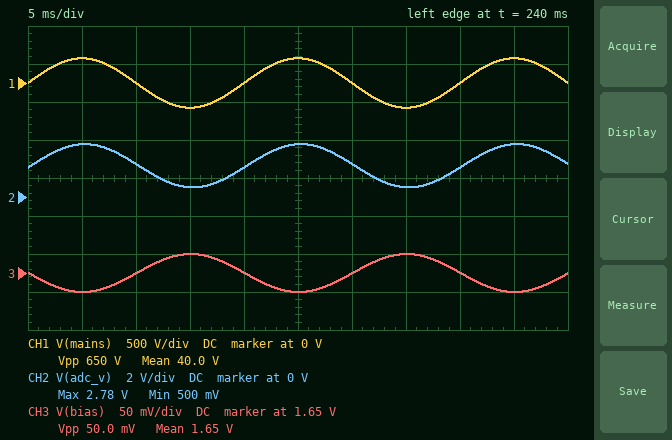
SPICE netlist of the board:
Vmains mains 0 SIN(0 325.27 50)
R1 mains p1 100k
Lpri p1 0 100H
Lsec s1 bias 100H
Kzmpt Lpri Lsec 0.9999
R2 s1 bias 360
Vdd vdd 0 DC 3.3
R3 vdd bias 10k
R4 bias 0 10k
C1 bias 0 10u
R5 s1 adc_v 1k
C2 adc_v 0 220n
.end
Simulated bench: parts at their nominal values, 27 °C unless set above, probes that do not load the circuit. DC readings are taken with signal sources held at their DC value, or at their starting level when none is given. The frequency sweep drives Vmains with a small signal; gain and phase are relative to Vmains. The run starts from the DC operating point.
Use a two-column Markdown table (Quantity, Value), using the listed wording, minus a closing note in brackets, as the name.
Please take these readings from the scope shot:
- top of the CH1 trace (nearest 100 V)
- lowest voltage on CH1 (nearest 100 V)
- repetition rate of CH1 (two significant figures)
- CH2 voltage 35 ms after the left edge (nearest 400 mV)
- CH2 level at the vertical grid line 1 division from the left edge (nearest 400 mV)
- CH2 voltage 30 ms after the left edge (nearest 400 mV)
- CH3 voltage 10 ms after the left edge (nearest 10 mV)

| Quantity | Value |
|---|---|
| top of the CH1 trace | 300 V |
| lowest voltage on CH1 | -300 V |
| repetition rate of CH1 | 50 Hz |
| CH2 voltage 35 ms after the left edge | 400 mV |
| CH2 level at the vertical grid line 1 division from the left edge | 2.8 V |
| CH2 voltage 30 ms after the left edge | 1.6 V |
| CH3 voltage 10 ms after the left edge | 1.65 V |
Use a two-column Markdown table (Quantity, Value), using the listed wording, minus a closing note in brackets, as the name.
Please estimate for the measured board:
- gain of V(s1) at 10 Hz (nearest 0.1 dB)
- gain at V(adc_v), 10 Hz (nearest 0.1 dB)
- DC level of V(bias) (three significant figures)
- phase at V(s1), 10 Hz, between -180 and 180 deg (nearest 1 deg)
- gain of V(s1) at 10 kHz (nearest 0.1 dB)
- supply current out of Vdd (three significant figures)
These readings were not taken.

| Quantity | Value |
|---|---|
| gain of V(s1) at 10 Hz | -49.1 dB |
| gain at V(adc_v), 10 Hz | -49.1 dB |
| DC level of V(bias) | 1.65 V |
| phase at V(s1), 10 Hz, between -180 and 180 deg | 3 deg |
| gain of V(s1) at 10 kHz | -51.6 dB |
| supply current out of Vdd | 165 µA |
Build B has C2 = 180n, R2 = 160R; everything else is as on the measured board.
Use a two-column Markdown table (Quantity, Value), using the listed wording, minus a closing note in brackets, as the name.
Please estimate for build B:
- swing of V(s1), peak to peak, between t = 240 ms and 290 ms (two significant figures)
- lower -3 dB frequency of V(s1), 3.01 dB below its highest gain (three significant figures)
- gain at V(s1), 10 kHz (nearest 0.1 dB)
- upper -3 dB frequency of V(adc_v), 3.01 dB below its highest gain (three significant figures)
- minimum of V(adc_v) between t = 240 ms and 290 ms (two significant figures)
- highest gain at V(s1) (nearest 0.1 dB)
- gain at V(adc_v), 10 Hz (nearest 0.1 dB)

| Quantity | Value |
|---|---|
| swing of V(s1), peak to peak, between t = 240 ms and 290 ms | 1.0 V |
| lower -3 dB frequency of V(s1), 3.01 dB below its highest gain | 248 mHz |
| gain at V(s1), 10 kHz | -57.2 dB |
| upper -3 dB frequency of V(adc_v), 3.01 dB below its highest gain | 767 Hz |
| minimum of V(adc_v) between t = 240 ms and 290 ms | 1.1 V |
| highest gain at V(s1) | -56.0 dB |
| gain at V(adc_v), 10 Hz | -56.1 dB |
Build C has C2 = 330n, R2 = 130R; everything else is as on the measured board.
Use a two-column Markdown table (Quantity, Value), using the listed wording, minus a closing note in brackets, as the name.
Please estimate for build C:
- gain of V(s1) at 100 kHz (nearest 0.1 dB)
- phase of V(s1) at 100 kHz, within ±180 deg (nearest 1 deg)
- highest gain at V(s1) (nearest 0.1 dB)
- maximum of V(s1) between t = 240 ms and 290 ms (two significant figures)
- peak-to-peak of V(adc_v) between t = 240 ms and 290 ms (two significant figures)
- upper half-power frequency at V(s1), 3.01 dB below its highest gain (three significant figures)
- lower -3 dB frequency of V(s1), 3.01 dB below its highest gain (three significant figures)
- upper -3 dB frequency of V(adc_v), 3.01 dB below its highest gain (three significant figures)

| Quantity | Value |
|---|---|
| gain of V(s1) at 100 kHz | -58.9 dB |
| phase of V(s1) at 100 kHz, within ±180 deg | -7 deg |
| highest gain at V(s1) | -57.9 dB |
| maximum of V(s1) between t = 240 ms and 290 ms | 2.1 V |
| peak-to-peak of V(adc_v) between t = 240 ms and 290 ms | 810 mV |
| upper half-power frequency at V(s1), 3.01 dB below its highest gain | 624 kHz |
| lower -3 dB frequency of V(s1), 3.01 dB below its highest gain | 201 mHz |
| upper -3 dB frequency of V(adc_v), 3.01 dB below its highest gain | 425 Hz |
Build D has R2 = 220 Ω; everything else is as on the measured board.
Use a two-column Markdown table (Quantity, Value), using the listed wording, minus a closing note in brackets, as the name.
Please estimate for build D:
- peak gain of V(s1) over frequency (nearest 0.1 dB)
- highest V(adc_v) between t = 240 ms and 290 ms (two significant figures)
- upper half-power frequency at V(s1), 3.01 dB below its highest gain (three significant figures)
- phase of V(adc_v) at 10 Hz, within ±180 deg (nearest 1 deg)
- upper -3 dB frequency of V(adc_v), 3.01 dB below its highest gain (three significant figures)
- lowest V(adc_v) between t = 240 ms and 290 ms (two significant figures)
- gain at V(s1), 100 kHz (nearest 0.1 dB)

| Quantity | Value |
|---|---|
| peak gain of V(s1) over frequency | -53.3 dB |
| highest V(adc_v) between t = 240 ms and 290 ms | 2.3 V |
| upper half-power frequency at V(s1), 3.01 dB below its highest gain | 499 kHz |
| phase of V(adc_v) at 10 Hz, within ±180 deg | 1 deg |
| upper -3 dB frequency of V(adc_v), 3.01 dB below its highest gain | 600 Hz |
| lowest V(adc_v) between t = 240 ms and 290 ms | 950 mV |
| gain at V(s1), 100 kHz | -55.0 dB |
